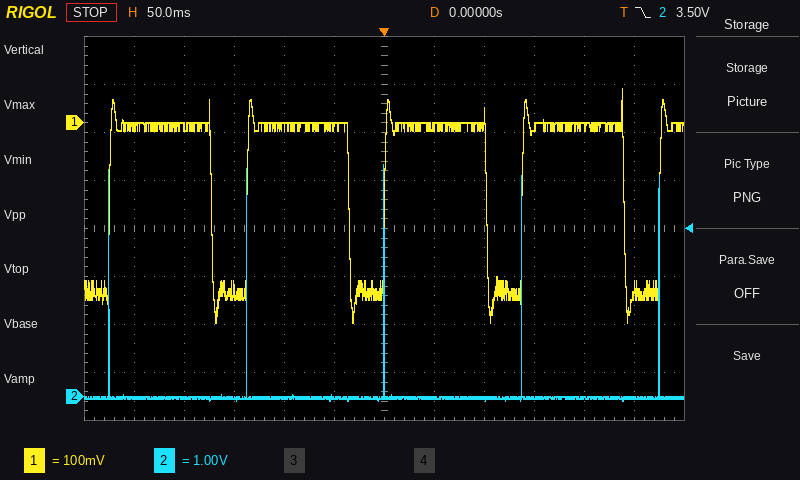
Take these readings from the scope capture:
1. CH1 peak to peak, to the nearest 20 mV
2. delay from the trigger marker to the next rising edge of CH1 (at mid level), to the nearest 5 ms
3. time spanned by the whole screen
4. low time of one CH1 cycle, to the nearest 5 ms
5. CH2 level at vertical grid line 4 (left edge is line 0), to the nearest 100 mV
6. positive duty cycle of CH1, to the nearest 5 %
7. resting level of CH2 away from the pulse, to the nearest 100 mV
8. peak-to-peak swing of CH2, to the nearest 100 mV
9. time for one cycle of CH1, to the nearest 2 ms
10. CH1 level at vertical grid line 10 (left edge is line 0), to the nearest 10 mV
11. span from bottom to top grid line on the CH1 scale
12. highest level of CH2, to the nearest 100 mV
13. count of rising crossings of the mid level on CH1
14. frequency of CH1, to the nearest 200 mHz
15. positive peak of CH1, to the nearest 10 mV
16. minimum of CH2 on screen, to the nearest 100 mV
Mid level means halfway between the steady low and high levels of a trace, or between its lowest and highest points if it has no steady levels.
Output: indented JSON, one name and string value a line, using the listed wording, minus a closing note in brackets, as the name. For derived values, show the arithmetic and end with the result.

{
  "CH1 peak to peak, to the nearest 20 mV": "480 mV",
  "delay from the trigger marker to the next rising edge of CH1 (at mid level), to the nearest 5 ms": "140 ms",
  "time spanned by the whole screen": "600 ms",
  "low time of one CH1 cycle, to the nearest 5 ms": "35 ms",
  "CH2 level at vertical grid line 4 (left edge is line 0), to the nearest 100 mV": "0.0 V",
  "positive duty cycle of CH1, to the nearest 5 %": "75 %",
  "resting level of CH2 away from the pulse, to the nearest 100 mV": "0.0 V",
  "peak-to-peak swing of CH2, to the nearest 100 mV": "4.8 V − (-100 mV) = 4.9 V",
  "time for one cycle of CH1, to the nearest 2 ms": "138 ms",
  "CH1 level at vertical grid line 10 (left edge is line 0), to the nearest 10 mV": "-10 mV",
  "span from bottom to top grid line on the CH1 scale": "800 mV",
  "highest level of CH2, to the nearest 100 mV": "4.8 V",
  "count of rising crossings of the mid level on CH1": "5",
  "frequency of CH1, to the nearest 200 mHz": "1 / 138 ms ≈ 7.2 Hz",
  "positive peak of CH1, to the nearest 10 mV": "70 mV",
  "minimum of CH2 on screen, to the nearest 100 mV": "-100 mV"
}
